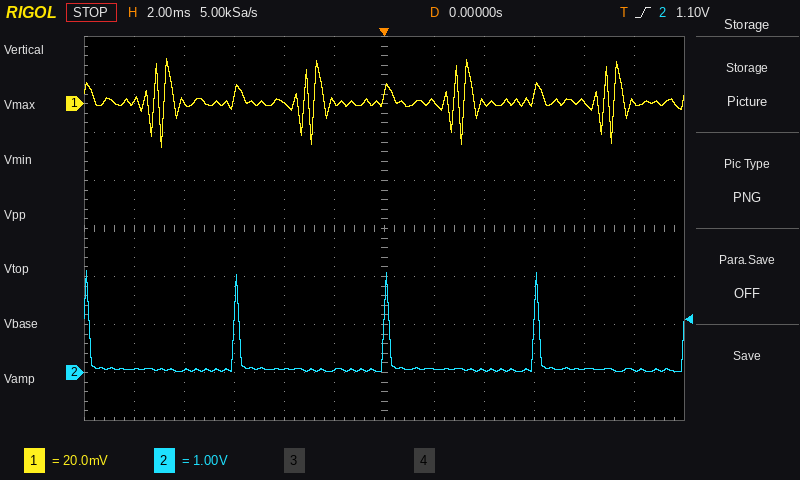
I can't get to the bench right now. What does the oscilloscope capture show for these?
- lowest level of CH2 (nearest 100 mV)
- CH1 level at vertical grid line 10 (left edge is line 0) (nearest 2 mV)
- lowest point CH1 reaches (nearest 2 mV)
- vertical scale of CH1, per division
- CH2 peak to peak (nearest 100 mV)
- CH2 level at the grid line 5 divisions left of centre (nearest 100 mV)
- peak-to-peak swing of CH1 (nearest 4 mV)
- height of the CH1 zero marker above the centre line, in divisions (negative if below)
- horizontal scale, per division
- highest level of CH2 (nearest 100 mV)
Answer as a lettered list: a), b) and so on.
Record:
a) 0.0 V
b) 0 mV
c) -18 mV
d) 20 mV
e) 2.1 V
f) 100 mV
g) 36 mV
h) +2.6 div
i) 2 ms
j) 2.1 V
